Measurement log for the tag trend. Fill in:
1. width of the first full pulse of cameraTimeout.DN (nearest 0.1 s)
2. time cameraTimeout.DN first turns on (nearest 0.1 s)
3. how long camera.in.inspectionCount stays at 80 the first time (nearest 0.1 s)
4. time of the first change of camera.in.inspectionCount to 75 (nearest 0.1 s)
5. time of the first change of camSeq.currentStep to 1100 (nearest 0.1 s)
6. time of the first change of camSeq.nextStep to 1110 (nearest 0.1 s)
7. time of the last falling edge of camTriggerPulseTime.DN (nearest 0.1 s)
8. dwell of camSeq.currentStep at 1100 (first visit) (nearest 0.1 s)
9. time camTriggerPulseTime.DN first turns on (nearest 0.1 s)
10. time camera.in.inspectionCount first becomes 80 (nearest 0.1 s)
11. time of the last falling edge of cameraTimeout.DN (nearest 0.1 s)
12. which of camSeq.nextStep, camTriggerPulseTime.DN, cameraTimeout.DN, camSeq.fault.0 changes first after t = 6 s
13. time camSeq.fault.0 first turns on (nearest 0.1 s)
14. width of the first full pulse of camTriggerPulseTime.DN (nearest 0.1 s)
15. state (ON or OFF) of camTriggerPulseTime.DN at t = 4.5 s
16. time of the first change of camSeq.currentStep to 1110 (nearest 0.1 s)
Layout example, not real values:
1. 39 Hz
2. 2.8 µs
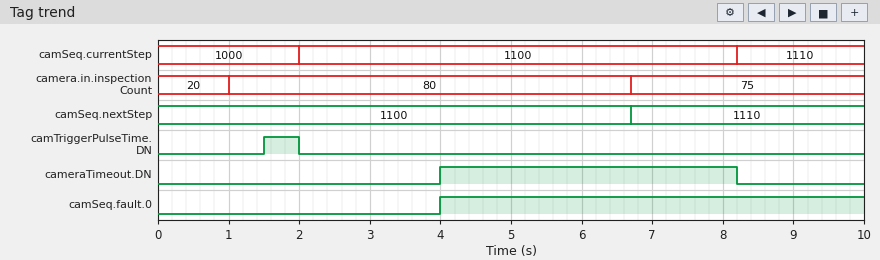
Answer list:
1. 4.2 s
2. 4.0 s
3. 5.7 s
4. 6.7 s
5. 2.0 s
6. 6.7 s
7. 2.0 s
8. 6.2 s
9. 1.5 s
10. 1.0 s
11. 8.2 s
12. camSeq.nextStep
13. 4.0 s
14. 0.5 s
15. OFF
16. 8.2 s
